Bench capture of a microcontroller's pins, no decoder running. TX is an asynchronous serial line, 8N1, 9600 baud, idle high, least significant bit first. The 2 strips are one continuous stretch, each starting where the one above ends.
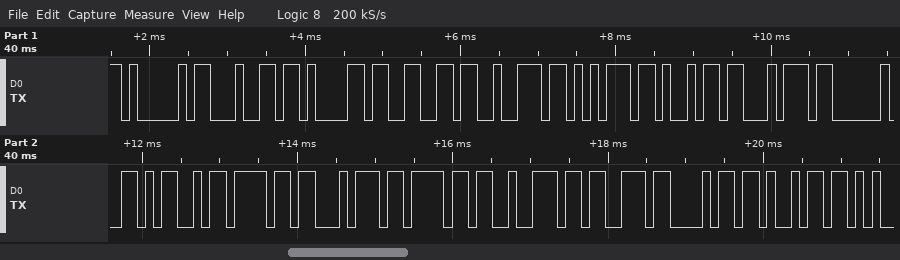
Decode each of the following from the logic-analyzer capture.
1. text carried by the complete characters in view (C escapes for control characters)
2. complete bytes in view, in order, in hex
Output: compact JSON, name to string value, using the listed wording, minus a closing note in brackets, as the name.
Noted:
{"text carried by the complete characters in view": "\"Adafruit Motorshi\"", "complete bytes in view, in order, in hex": "0x41 0x64 0x61 0x66 0x72 0x75 0x69 0x74 0x20 0x4D 0x6F 0x74 0x6F 0x72 0x73 0x68 0x69"}
